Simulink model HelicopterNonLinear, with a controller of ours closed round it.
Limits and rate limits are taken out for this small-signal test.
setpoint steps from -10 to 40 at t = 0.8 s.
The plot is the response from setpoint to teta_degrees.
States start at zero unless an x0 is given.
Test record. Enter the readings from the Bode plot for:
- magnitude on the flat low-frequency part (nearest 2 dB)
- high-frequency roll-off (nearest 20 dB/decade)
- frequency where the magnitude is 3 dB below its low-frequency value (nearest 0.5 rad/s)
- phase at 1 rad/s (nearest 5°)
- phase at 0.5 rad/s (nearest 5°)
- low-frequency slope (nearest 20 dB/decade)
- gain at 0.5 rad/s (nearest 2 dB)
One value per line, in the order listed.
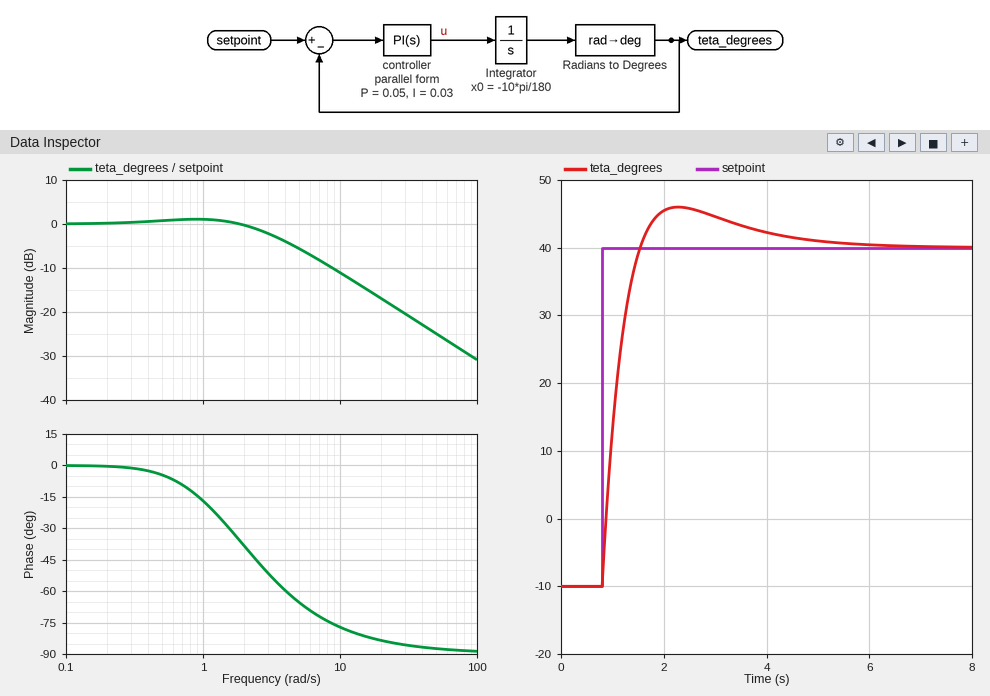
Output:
0 dB
-20 dB/decade
3.5 rad/s
-15°
-5°
0 dB/decade
0 dB
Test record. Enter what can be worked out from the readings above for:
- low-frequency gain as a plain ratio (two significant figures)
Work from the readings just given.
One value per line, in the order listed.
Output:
1.0
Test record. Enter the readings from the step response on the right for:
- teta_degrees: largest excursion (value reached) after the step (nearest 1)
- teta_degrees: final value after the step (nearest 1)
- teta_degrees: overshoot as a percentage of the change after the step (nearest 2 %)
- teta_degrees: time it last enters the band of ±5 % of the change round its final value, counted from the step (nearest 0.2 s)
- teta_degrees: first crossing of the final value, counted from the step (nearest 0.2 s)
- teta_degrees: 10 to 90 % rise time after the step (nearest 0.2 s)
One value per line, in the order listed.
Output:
46
40
12 %
3.0 s
0.8 s
0.6 s
